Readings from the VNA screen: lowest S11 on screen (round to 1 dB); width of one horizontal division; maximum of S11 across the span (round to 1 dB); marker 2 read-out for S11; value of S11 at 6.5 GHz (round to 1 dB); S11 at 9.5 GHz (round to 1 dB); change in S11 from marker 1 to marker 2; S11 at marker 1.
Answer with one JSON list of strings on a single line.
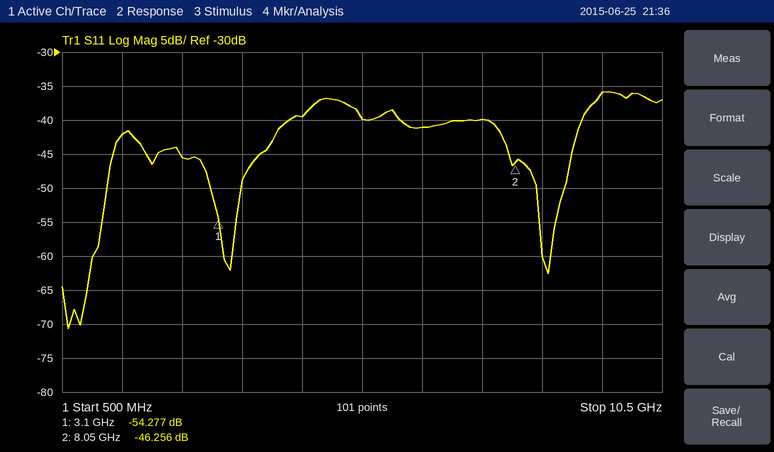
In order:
["-71 dB", "1 GHz", "-36 dB", "-46.256 dB", "-41 dB", "-36 dB", "8.021 dB", "-54.277 dB"]
